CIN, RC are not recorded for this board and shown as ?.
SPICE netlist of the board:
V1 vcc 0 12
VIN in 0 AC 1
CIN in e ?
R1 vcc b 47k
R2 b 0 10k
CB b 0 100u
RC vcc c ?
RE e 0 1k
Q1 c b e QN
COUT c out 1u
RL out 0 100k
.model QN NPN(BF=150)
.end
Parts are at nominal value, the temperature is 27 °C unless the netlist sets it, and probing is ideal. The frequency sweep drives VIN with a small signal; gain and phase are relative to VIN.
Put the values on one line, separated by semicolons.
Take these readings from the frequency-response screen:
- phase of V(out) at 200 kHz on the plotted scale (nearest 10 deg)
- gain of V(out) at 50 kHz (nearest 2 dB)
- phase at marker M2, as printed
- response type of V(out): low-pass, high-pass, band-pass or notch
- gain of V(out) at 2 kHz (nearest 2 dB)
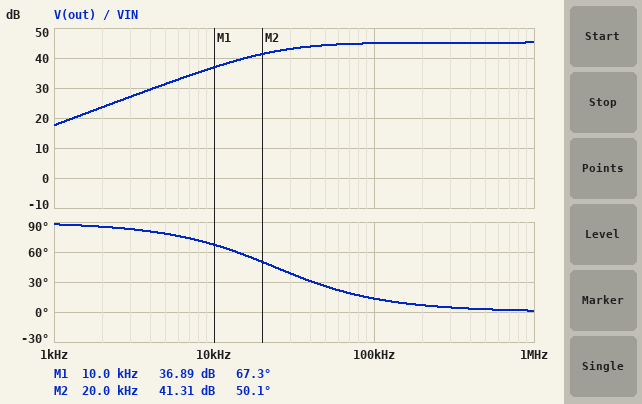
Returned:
10 deg; 44 dB; 50.1 deg; high-pass; 24 dB
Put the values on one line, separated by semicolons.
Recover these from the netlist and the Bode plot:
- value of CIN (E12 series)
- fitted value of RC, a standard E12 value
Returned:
330 nF; 3.9 kΩ
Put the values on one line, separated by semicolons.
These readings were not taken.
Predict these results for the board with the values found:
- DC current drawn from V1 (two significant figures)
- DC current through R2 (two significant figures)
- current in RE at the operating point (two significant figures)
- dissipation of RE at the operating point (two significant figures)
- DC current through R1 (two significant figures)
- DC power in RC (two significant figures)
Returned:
1.5 mA; 200 µA; 1.3 mA; 1.6 mW; 210 µA; 6.1 mW
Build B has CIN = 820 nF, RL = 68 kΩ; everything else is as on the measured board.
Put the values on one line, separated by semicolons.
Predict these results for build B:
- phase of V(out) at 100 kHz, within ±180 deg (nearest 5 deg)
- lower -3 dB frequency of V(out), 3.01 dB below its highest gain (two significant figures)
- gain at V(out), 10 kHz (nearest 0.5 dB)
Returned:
5 deg; 9.6 kHz; 42.0 dB
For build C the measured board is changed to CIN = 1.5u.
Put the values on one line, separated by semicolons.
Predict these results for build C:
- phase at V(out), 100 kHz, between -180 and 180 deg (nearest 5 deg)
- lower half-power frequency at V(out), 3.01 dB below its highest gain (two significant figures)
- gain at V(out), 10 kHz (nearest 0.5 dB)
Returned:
5 deg; 5.3 kHz; 44.0 dB
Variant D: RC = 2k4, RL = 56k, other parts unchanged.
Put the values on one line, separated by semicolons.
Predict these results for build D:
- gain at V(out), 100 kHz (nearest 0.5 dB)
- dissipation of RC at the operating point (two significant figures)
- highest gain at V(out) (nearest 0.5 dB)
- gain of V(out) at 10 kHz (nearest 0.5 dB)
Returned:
40.5 dB; 3.7 mW; 41.0 dB; 32.5 dB
